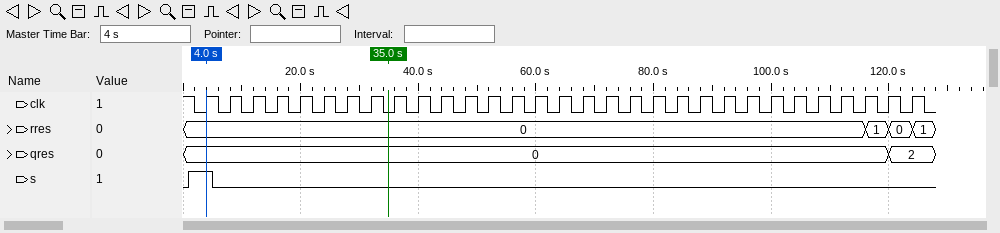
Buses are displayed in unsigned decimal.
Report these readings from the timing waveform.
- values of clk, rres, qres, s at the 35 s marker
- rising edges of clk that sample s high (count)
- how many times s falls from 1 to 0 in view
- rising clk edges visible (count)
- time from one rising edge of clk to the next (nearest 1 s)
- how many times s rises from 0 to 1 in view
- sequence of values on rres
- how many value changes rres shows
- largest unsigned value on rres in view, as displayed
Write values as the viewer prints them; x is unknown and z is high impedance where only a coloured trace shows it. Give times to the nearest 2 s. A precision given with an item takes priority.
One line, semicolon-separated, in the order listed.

clk=0, rres=0, qres=0, s=0; 1; 1; 31; 4 s; 1; 0, 1, 0, 1; 3; 1
